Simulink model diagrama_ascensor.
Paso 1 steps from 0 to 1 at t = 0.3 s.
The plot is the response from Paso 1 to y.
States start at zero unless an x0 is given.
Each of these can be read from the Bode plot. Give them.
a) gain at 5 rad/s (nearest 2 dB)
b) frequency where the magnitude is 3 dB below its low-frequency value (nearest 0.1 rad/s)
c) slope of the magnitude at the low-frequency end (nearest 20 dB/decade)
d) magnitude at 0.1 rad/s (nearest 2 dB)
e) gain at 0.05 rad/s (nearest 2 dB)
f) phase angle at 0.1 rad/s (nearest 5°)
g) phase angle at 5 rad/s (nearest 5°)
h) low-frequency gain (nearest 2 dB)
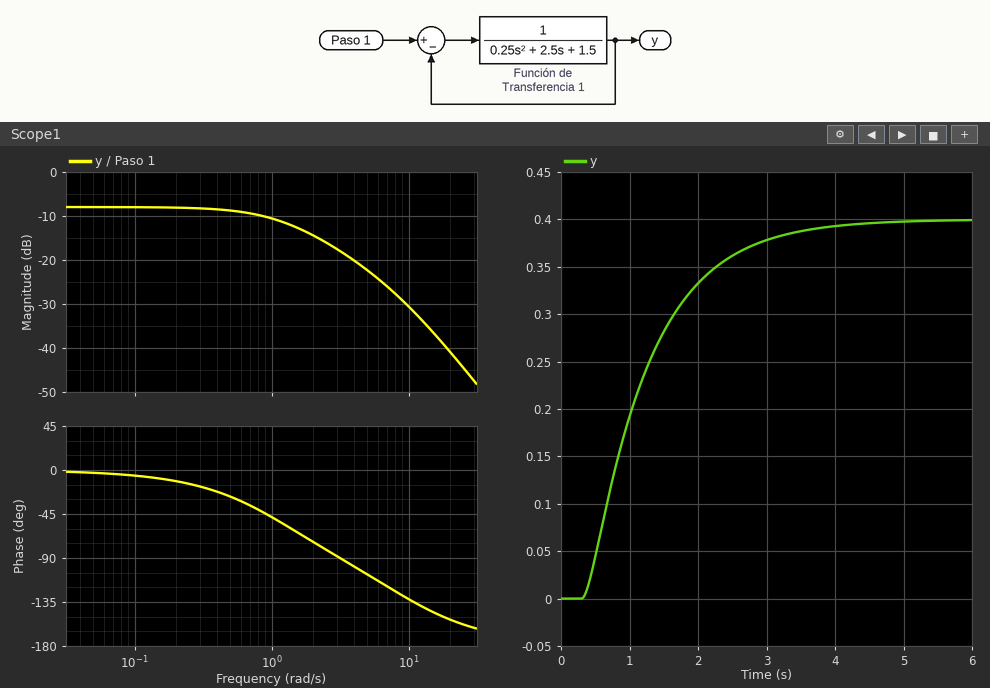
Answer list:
-22 dB
1.1 rad/s
0 dB/decade
-8 dB
-8 dB
-5°
-105°
-8 dB
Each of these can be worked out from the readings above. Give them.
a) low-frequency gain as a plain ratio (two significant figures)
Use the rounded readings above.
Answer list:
0.40
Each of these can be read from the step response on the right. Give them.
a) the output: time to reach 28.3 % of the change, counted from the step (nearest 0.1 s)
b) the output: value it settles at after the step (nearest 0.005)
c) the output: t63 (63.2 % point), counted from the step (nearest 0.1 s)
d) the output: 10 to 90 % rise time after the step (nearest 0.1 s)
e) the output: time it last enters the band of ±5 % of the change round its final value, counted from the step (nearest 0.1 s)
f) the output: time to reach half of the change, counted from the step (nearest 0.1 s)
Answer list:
0.4 s
0.400
1.0 s
2.0 s
2.8 s
0.7 s
